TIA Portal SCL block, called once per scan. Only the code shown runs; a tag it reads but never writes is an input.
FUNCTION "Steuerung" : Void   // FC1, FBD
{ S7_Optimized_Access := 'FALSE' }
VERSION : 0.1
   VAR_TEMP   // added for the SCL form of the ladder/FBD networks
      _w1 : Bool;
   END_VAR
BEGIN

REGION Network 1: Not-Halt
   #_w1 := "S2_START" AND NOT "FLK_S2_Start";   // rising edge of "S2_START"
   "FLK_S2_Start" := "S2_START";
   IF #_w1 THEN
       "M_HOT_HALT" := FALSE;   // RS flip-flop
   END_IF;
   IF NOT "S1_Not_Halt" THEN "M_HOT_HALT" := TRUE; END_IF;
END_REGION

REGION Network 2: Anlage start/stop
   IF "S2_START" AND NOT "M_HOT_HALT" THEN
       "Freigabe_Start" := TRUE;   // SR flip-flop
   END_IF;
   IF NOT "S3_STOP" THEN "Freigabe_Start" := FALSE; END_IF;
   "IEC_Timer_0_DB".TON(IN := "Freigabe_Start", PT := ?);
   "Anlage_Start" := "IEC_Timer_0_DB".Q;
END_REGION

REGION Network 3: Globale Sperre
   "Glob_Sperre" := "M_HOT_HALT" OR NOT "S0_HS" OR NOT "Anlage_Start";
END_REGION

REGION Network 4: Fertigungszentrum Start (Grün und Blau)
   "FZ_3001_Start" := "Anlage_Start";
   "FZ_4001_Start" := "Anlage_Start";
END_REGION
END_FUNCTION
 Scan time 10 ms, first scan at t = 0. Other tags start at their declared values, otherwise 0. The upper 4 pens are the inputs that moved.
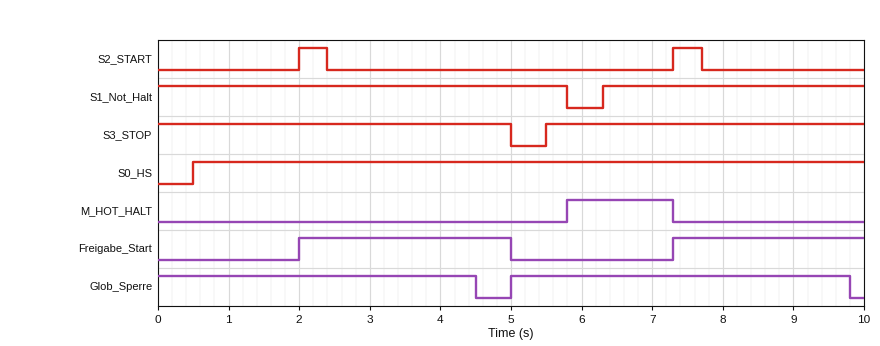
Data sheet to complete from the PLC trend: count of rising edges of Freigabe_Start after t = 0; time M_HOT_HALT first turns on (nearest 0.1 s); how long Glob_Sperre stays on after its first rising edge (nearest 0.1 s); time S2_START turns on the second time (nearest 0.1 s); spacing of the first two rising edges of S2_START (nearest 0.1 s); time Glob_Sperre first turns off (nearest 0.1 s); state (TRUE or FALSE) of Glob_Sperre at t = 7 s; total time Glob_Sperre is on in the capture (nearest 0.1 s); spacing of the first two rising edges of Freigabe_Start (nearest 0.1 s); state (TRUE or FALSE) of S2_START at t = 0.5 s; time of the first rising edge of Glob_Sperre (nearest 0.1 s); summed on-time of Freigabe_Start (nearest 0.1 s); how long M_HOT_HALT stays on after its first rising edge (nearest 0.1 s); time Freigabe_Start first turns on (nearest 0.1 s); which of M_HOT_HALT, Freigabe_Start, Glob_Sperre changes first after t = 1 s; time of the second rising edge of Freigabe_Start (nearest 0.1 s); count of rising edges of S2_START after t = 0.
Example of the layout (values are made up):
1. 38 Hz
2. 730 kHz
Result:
1. 2
2. 5.8 s
3. 4.8 s
4. 7.3 s
5. 5.3 s
6. 4.5 s
7. TRUE
8. 9.3 s
9. 5.3 s
10. FALSE
11. 5.0 s
12. 5.7 s
13. 1.5 s
14. 2.0 s
15. Freigabe_Start
16. 7.3 s
17. 2
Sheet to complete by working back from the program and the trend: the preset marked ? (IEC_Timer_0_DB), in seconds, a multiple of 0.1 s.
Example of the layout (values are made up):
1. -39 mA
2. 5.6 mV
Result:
1. 2.5 s
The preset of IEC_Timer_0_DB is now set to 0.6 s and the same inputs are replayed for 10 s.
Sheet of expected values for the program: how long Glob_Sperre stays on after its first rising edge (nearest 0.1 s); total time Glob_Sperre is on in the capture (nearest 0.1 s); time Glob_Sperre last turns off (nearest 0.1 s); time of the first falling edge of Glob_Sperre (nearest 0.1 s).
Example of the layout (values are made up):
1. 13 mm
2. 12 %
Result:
1. 2.9 s
2. 5.5 s
3. 7.9 s
4. 2.6 s
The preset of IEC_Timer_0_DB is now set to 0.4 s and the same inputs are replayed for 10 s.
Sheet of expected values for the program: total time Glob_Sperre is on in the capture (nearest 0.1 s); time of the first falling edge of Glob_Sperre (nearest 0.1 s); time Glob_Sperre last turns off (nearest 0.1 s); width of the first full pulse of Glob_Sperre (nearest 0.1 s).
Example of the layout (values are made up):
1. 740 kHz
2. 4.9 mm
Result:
1. 5.1 s
2. 2.4 s
3. 7.7 s
4. 2.7 s
